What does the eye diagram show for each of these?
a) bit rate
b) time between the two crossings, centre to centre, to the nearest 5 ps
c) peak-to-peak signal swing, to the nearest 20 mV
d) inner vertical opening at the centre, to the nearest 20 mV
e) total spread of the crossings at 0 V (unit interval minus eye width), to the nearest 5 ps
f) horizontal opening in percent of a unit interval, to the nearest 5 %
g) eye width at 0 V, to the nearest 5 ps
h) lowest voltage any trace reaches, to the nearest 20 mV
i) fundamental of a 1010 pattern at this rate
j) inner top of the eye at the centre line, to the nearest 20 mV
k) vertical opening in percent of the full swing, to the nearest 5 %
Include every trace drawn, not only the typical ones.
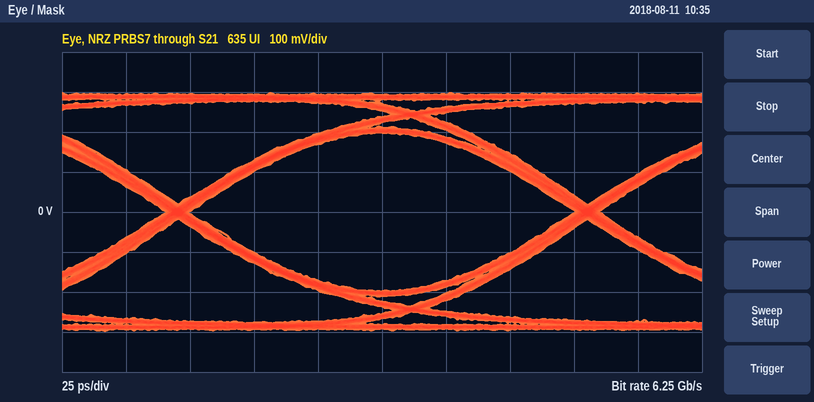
6.25 Gb/s
160 ps
600 mV
400 mV
10 ps
95 %
150 ps
-300 mV
3.125 GHz
200 mV
65 %
